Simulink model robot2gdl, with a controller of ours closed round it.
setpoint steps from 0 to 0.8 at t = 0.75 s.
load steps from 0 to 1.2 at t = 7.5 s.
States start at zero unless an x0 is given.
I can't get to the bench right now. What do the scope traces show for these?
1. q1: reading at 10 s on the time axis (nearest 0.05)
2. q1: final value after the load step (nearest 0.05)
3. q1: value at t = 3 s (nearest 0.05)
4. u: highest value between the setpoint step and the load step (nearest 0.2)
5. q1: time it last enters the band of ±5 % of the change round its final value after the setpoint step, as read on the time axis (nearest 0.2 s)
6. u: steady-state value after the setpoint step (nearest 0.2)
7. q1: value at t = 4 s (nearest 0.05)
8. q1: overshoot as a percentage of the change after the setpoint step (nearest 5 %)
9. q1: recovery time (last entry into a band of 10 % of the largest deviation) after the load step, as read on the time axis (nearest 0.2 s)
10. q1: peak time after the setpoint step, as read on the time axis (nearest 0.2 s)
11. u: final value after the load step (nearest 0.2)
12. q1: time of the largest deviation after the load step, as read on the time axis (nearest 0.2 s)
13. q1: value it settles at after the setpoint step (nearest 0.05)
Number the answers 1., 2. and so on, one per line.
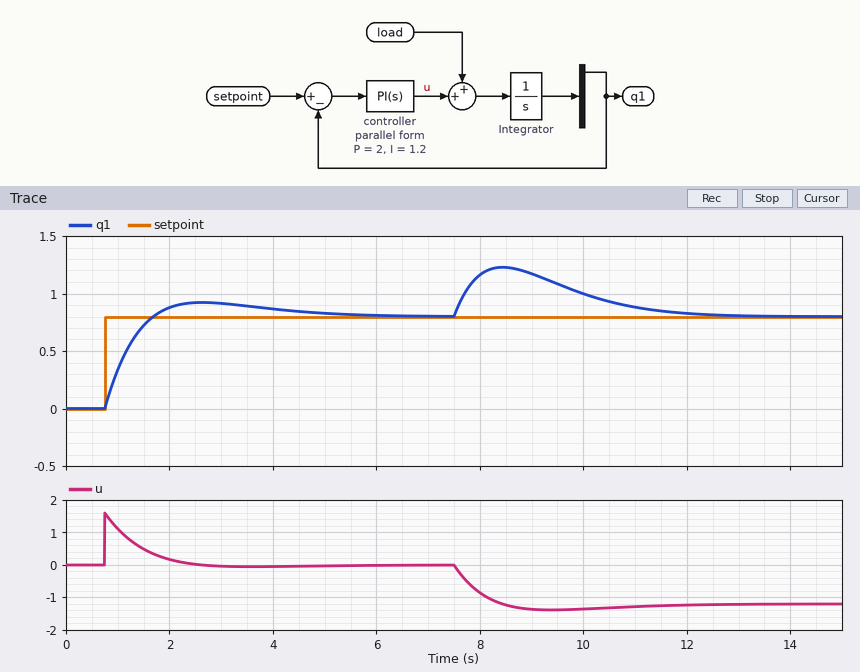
1. 1.00
2. 0.80
3. 0.90
4. 1.6
5. 4.6 s
6. 0.0
7. 0.85
8. 15 %
9. 11.6 s
10. 2.6 s
11. -1.2
12. 8.4 s
13. 0.80
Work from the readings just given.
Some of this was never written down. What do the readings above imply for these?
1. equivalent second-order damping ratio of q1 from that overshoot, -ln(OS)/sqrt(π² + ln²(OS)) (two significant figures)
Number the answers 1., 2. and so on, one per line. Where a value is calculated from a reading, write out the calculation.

1. ln(0.15) = -1.897; 1.897 / sqrt(9.870 + 3.599) = 0.52
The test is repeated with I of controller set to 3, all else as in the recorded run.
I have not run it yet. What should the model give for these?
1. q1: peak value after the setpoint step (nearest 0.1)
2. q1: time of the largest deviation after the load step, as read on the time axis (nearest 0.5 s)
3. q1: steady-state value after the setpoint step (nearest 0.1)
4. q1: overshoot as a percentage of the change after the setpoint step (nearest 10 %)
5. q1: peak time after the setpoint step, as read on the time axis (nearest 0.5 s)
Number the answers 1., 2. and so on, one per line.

1. 1.0
2. 8.0 s
3. 0.8
4. 30 %
5. 2.0 s
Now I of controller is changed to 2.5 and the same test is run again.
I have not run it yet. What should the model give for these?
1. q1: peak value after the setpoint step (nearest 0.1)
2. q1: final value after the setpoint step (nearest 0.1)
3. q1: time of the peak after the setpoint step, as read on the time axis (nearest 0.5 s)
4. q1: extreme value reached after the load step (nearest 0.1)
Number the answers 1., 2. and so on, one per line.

1. 1.0
2. 0.8
3. 2.0 s
4. 1.2
